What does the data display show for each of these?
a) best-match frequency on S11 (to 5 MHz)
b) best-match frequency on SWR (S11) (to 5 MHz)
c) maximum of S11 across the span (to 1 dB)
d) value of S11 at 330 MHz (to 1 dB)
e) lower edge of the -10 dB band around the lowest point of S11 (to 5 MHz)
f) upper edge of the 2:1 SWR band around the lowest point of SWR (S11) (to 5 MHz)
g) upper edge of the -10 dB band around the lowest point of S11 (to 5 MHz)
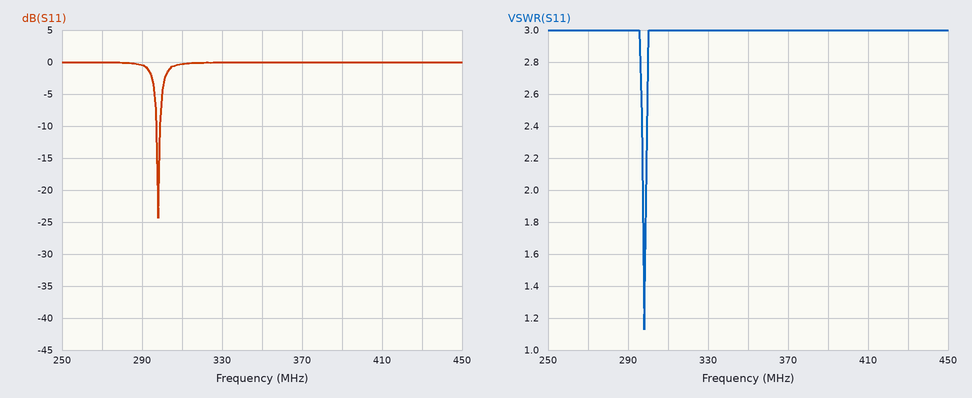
300 MHz
300 MHz
0 dB
0 dB
295 MHz
300 MHz
300 MHz
